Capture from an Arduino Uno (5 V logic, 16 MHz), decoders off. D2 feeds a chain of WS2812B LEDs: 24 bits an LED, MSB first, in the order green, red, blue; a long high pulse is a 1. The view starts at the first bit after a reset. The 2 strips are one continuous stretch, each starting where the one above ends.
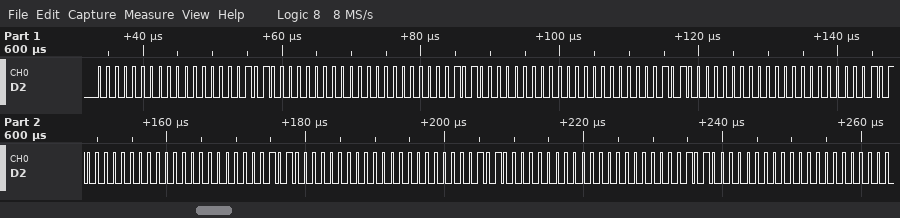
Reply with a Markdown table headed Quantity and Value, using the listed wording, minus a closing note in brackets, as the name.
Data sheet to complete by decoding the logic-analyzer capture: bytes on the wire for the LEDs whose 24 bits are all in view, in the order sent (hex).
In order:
| Quantity | Value |
|---|---|
| bytes on the wire for the LEDs whose 24 bits are all in view, in the order sent | 00 00 50 00 00 50 00 00 50 00 00 50 00 00 50 00 00 50 00 00 50 |
